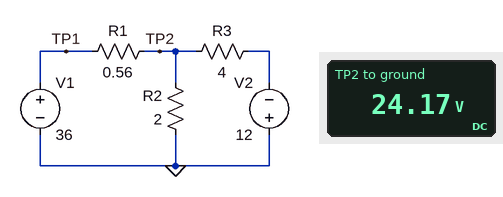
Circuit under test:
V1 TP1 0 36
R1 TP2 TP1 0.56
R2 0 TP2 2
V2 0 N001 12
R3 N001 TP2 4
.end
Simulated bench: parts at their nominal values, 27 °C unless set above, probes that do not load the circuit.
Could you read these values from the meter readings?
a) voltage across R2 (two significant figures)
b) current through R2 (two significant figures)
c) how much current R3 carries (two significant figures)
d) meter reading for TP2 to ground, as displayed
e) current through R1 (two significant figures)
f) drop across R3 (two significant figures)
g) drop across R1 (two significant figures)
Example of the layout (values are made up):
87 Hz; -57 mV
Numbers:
24 V; 12 A; 9.0 A; 24.17 V; 21 A; 36 V; 12 V
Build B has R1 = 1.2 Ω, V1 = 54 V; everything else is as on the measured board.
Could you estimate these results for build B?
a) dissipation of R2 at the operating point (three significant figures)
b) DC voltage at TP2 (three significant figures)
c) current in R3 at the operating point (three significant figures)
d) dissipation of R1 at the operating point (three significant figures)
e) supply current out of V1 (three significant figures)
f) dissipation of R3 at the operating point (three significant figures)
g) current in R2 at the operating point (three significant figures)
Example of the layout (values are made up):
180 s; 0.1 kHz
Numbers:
352 W; 26.5 V; 9.63 A; 629 W; 22.9 A; 371 W; 13.3 A
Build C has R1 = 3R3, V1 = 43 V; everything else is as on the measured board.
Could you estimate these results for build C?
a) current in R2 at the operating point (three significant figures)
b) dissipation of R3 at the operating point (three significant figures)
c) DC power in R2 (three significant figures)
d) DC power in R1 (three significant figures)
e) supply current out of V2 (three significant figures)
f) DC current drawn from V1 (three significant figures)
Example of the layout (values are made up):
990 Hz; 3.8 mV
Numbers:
4.76 A; 116 W; 45.4 W; 340 W; 5.38 A; 10.1 A
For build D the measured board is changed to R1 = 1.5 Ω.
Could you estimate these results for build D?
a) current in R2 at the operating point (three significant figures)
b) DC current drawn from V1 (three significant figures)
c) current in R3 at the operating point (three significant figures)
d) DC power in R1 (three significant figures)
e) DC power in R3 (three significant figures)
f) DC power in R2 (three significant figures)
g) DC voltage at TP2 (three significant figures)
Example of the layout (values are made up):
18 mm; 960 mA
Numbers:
7.41 A; 14.1 A; 6.71 A; 299 W; 180 W; 110 W; 14.8 V
